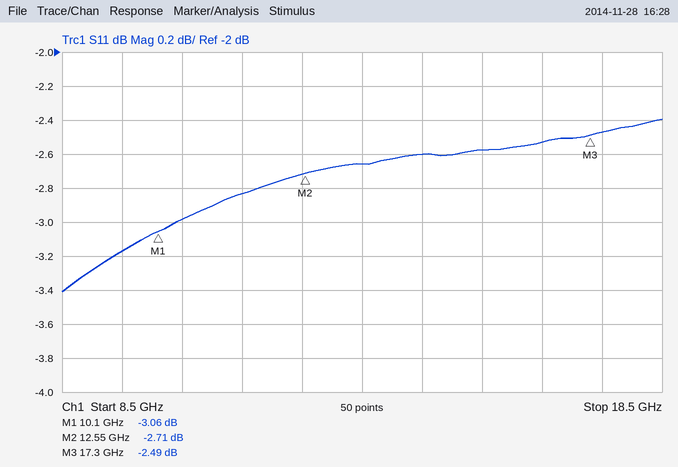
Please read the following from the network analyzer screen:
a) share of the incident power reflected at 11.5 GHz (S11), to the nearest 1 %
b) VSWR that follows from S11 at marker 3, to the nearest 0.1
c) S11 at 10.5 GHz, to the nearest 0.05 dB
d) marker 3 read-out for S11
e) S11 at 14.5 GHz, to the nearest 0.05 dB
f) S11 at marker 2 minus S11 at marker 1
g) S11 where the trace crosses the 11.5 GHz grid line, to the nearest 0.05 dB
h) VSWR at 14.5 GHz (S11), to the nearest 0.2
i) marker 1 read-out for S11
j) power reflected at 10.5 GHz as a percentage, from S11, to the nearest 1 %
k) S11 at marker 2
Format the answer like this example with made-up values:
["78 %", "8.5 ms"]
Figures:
["52 %", "7.0", "-3.00 dB", "-2.49 dB", "-2.60 dB", "0.35 dB", "-2.85 dB", "6.8", "-3.06 dB", "50 %", "-2.71 dB"]
